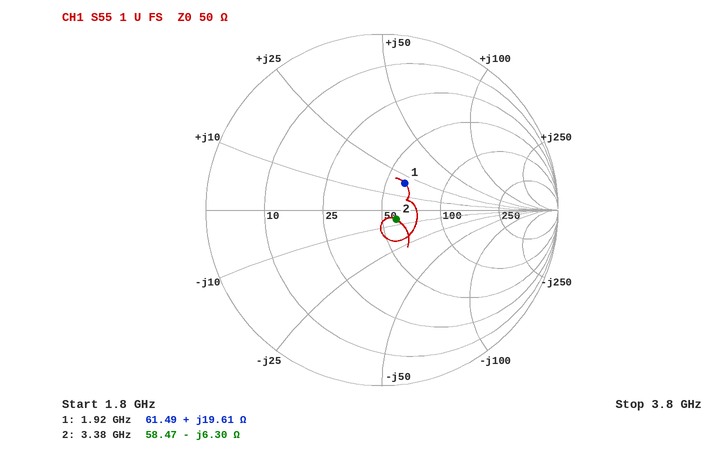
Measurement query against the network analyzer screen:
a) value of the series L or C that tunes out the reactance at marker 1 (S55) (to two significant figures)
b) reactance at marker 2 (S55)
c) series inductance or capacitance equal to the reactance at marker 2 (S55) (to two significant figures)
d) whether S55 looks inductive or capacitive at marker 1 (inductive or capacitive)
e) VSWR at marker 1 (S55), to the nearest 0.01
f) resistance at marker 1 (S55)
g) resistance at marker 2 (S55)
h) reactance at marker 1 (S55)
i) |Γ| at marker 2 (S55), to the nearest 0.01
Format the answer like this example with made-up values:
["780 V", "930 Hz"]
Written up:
["4.2 pF", "-6.30 Ω", "7.5 pF", "inductive", "1.50", "61.49 Ω", "58.47 Ω", "+19.61 Ω", "0.10"]
